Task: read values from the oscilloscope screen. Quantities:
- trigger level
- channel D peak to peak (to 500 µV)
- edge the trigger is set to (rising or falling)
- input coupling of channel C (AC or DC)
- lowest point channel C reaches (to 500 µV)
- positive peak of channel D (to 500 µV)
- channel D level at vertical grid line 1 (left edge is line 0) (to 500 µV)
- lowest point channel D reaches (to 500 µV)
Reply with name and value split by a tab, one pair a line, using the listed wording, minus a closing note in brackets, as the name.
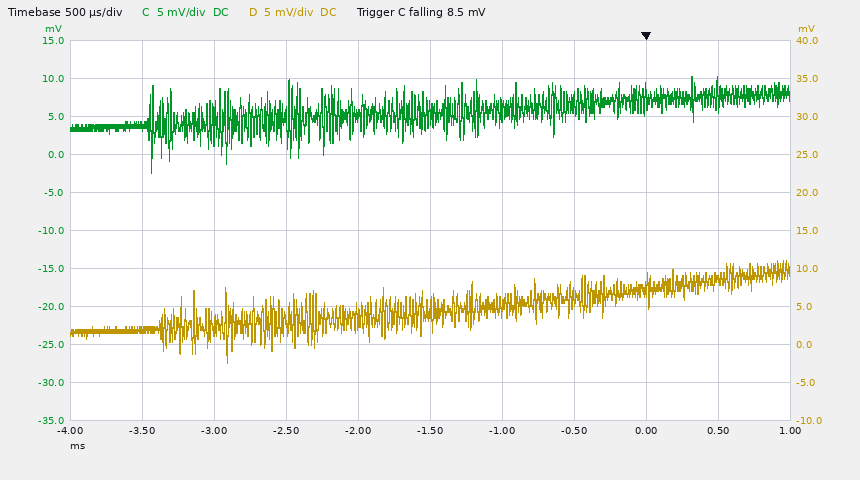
trigger level	8.5 mV
channel D peak to peak	13.5 mV
edge the trigger is set to	falling
input coupling of channel C	DC
lowest point channel C reaches	-2.5 mV
positive peak of channel D	11.0 mV
channel D level at vertical grid line 1 (left edge is line 0)	2.0 mV
lowest point channel D reaches	-2.5 mV
